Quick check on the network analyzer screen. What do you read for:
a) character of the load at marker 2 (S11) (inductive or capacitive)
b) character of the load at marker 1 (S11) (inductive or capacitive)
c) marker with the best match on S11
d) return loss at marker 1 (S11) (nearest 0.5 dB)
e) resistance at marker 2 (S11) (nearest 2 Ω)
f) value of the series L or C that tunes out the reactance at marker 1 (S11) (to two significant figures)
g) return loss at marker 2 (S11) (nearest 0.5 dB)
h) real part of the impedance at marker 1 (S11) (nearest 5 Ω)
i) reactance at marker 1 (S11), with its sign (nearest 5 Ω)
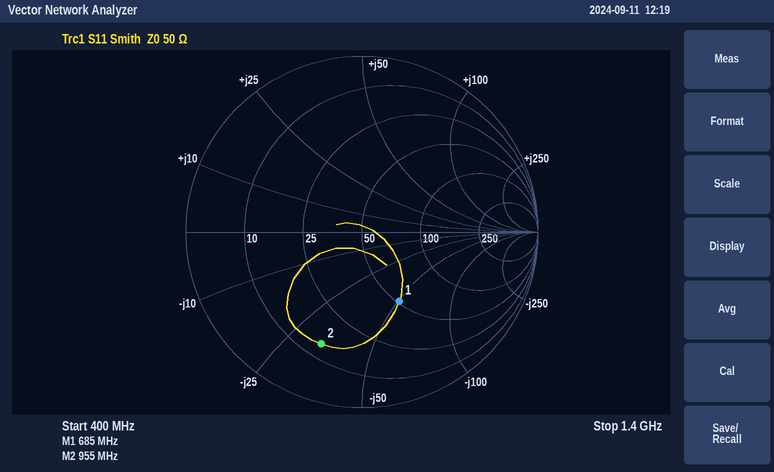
capacitive
capacitive
marker 1
7.0 dB
14 Ω
12 nH
3.5 dB
50 Ω
-50 Ω
